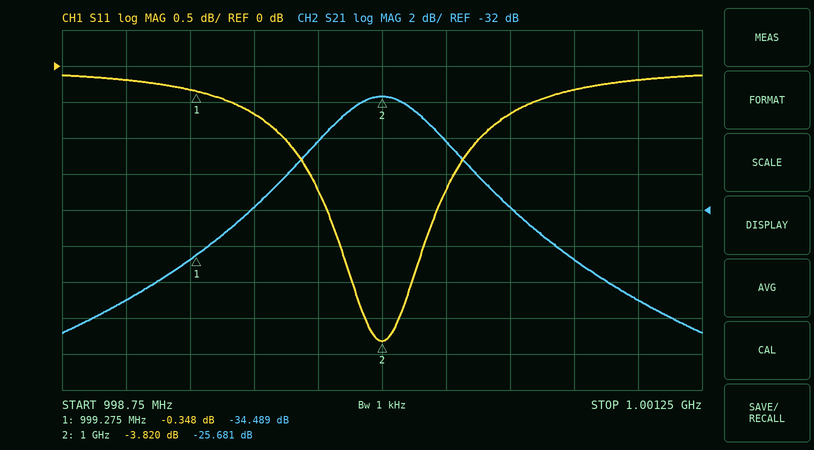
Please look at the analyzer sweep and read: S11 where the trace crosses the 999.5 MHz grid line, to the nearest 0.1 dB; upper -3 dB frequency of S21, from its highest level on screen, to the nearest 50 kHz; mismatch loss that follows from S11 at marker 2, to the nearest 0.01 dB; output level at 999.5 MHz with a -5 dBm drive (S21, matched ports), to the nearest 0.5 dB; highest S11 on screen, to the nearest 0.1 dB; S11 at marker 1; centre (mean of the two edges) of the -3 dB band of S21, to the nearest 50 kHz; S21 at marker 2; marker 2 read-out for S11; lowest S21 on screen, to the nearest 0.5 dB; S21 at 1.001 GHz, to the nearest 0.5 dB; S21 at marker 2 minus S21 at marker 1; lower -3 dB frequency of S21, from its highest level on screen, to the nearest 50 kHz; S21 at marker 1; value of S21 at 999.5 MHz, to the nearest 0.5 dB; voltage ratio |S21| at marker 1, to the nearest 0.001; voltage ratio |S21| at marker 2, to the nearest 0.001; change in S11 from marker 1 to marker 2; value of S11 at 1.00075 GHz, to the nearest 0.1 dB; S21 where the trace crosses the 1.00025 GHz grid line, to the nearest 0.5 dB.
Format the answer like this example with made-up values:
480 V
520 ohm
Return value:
-0.7 dB
1.00030 GHz
2.33 dB
-37.0 dBm
-0.1 dB
-0.348 dB
1.00000 GHz
-25.681 dB
-3.820 dB
-39.0 dB
-37.0 dB
8.808 dB
999.70 MHz
-34.489 dB
-32.0 dB
0.019
0.052
-3.472 dB
-0.3 dB
-28.0 dB
